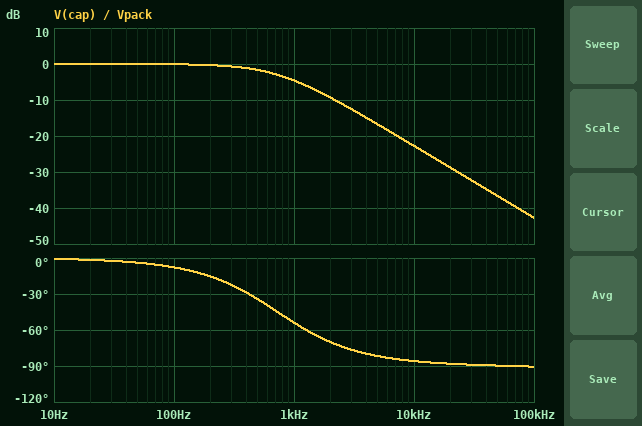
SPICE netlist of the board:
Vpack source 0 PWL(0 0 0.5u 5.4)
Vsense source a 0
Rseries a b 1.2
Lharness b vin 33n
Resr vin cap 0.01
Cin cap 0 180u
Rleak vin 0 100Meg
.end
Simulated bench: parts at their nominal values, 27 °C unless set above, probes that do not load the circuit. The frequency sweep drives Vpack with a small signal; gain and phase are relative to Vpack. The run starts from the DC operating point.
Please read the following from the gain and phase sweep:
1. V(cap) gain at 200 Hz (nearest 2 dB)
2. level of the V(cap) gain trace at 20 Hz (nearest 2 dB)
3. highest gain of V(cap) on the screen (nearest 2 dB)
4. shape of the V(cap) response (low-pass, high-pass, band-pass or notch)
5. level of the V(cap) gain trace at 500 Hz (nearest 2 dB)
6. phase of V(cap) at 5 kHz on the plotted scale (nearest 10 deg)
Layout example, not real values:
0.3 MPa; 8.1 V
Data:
0 dB; 0 dB; 0 dB; low-pass; -2 dB; -80 deg
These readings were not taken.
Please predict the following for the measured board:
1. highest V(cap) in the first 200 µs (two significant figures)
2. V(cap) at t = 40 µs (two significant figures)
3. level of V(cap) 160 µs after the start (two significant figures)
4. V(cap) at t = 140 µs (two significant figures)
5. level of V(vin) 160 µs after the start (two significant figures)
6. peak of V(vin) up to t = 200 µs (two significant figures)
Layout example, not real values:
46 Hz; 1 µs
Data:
3.2 V; 900 mV; 2.8 V; 2.6 V; 2.8 V; 3.3 V
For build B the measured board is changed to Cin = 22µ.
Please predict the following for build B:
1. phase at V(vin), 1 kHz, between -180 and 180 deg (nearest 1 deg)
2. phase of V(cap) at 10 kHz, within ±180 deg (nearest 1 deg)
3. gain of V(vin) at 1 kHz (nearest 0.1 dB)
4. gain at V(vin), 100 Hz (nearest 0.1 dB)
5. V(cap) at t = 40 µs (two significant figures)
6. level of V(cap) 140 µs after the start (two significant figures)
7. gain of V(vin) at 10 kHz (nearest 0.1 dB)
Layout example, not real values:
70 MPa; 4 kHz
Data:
-9 deg; -59 deg; -0.1 dB; 0 dB; 4.2 V; 5.4 V; -5.8 dB
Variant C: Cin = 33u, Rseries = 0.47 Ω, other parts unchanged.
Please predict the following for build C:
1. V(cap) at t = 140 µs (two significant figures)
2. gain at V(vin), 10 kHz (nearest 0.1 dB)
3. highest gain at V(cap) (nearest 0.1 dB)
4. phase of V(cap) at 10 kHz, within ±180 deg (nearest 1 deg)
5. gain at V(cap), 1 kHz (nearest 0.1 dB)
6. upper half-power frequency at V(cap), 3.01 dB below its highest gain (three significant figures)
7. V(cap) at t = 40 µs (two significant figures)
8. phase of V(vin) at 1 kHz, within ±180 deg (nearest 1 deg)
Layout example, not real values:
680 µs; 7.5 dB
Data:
5.4 V; -3.0 dB; 0 dB; -45 deg; 0 dB; 10.1 kHz; 5.0 V; -6 deg
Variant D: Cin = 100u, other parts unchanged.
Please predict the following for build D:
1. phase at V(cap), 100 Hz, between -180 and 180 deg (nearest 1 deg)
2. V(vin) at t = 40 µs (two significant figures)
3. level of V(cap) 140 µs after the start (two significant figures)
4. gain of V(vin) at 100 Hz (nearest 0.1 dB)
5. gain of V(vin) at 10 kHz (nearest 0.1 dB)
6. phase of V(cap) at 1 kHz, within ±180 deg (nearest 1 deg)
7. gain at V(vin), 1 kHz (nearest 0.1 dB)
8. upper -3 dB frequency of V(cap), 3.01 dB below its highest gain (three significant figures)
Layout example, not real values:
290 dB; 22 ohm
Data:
-4 deg; 1.5 V; 3.7 V; 0 dB; -17.7 dB; -37 deg; -2.0 dB; 1.32 kHz
